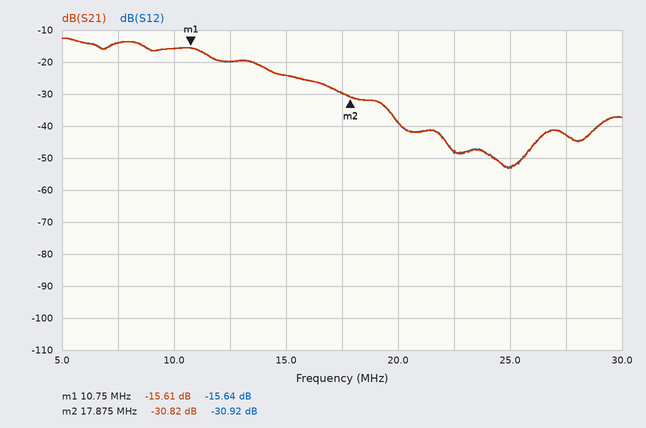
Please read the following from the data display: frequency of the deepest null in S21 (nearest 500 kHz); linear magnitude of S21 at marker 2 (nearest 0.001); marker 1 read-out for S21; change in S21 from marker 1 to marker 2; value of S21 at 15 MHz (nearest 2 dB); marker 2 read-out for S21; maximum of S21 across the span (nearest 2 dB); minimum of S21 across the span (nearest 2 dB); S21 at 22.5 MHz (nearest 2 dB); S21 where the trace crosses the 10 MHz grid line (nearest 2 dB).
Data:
25.0 MHz
0.029
-15.61 dB
-15.21 dB
-24 dB
-30.82 dB
-12 dB
-54 dB
-48 dB
-16 dB
